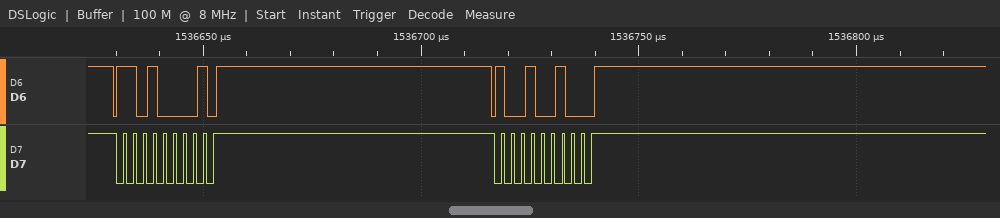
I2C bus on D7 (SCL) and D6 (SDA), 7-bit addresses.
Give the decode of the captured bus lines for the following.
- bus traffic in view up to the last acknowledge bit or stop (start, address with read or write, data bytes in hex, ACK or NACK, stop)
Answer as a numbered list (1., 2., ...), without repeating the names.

1. start, address 68 write NACK, stop, start, address 49 write ACK, stop
